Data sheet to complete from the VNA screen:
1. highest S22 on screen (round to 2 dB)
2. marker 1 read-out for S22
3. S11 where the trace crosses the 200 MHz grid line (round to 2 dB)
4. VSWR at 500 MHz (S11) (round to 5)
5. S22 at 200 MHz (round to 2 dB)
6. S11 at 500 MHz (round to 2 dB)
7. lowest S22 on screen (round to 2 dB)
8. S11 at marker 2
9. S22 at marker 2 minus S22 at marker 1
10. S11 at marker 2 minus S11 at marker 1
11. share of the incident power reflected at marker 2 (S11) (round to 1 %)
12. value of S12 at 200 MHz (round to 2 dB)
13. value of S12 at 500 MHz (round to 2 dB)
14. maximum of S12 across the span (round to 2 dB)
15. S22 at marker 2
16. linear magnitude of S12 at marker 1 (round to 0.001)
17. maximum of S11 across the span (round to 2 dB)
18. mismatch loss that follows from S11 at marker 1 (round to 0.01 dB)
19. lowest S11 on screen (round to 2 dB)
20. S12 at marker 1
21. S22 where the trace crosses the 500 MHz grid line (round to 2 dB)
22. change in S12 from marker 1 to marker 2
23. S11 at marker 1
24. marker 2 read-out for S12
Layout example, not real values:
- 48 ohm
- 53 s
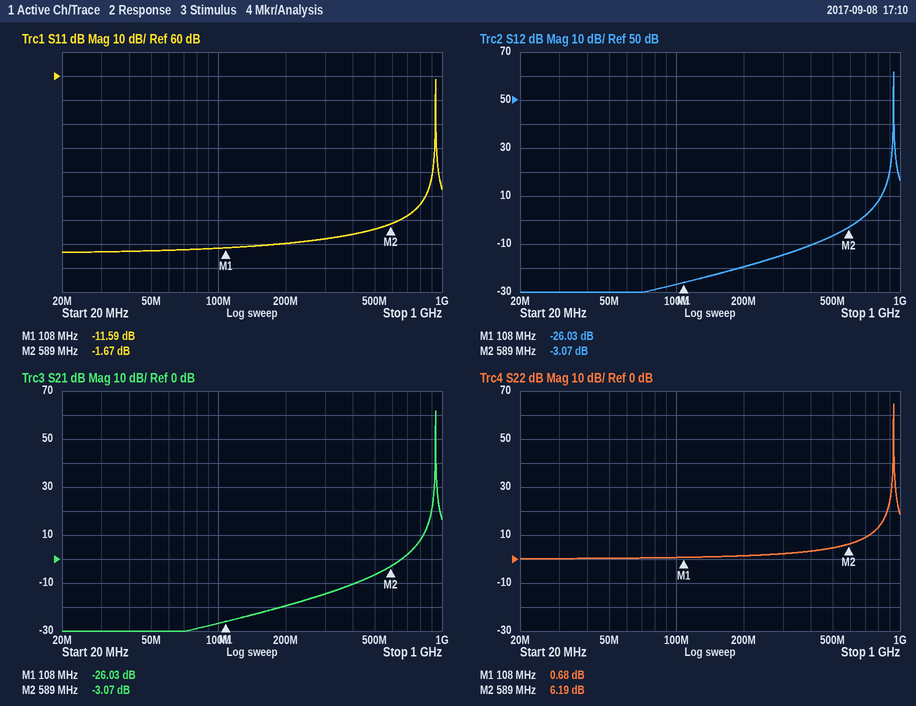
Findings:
- 64 dB
- 0.68 dB
- -10 dB
- 5
- 2 dB
- -4 dB
- 0 dB
- -1.67 dB
- 5.51 dB
- 9.92 dB
- 68 %
- -20 dB
- -6 dB
- 62 dB
- 6.19 dB
- 0.050
- 58 dB
- 0.31 dB
- -14 dB
- -26.03 dB
- 4 dB
- 22.96 dB
- -11.59 dB
- -3.07 dB
